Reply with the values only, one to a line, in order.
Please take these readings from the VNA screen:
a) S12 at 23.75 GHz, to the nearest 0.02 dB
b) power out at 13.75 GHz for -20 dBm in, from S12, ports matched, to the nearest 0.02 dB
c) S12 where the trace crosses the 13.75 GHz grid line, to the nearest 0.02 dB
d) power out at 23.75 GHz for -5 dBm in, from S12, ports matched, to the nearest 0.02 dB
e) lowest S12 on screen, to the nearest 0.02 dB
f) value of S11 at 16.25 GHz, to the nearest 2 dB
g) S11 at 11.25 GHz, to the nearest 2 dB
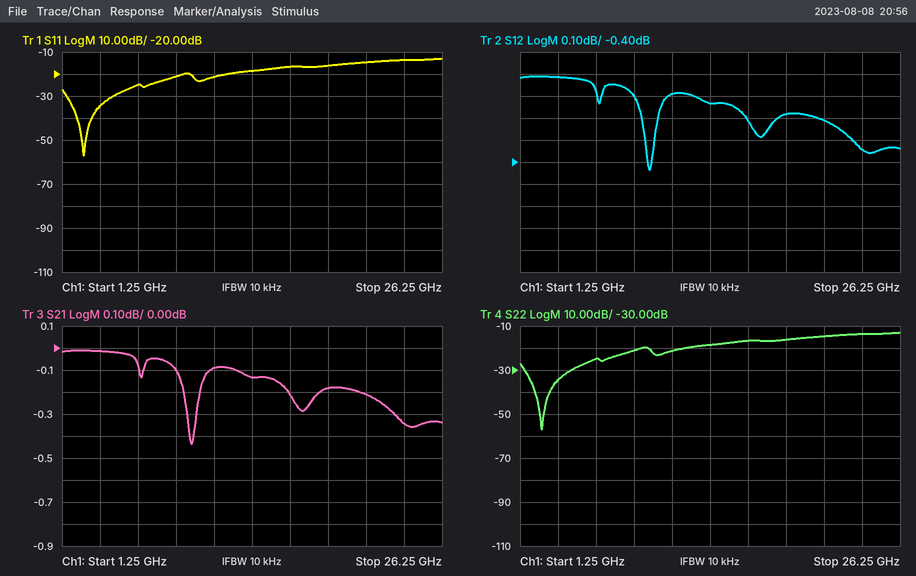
-0.34 dB
-20.14 dBm
-0.14 dB
-5.34 dBm
-0.44 dB
-16 dB
-22 dB
